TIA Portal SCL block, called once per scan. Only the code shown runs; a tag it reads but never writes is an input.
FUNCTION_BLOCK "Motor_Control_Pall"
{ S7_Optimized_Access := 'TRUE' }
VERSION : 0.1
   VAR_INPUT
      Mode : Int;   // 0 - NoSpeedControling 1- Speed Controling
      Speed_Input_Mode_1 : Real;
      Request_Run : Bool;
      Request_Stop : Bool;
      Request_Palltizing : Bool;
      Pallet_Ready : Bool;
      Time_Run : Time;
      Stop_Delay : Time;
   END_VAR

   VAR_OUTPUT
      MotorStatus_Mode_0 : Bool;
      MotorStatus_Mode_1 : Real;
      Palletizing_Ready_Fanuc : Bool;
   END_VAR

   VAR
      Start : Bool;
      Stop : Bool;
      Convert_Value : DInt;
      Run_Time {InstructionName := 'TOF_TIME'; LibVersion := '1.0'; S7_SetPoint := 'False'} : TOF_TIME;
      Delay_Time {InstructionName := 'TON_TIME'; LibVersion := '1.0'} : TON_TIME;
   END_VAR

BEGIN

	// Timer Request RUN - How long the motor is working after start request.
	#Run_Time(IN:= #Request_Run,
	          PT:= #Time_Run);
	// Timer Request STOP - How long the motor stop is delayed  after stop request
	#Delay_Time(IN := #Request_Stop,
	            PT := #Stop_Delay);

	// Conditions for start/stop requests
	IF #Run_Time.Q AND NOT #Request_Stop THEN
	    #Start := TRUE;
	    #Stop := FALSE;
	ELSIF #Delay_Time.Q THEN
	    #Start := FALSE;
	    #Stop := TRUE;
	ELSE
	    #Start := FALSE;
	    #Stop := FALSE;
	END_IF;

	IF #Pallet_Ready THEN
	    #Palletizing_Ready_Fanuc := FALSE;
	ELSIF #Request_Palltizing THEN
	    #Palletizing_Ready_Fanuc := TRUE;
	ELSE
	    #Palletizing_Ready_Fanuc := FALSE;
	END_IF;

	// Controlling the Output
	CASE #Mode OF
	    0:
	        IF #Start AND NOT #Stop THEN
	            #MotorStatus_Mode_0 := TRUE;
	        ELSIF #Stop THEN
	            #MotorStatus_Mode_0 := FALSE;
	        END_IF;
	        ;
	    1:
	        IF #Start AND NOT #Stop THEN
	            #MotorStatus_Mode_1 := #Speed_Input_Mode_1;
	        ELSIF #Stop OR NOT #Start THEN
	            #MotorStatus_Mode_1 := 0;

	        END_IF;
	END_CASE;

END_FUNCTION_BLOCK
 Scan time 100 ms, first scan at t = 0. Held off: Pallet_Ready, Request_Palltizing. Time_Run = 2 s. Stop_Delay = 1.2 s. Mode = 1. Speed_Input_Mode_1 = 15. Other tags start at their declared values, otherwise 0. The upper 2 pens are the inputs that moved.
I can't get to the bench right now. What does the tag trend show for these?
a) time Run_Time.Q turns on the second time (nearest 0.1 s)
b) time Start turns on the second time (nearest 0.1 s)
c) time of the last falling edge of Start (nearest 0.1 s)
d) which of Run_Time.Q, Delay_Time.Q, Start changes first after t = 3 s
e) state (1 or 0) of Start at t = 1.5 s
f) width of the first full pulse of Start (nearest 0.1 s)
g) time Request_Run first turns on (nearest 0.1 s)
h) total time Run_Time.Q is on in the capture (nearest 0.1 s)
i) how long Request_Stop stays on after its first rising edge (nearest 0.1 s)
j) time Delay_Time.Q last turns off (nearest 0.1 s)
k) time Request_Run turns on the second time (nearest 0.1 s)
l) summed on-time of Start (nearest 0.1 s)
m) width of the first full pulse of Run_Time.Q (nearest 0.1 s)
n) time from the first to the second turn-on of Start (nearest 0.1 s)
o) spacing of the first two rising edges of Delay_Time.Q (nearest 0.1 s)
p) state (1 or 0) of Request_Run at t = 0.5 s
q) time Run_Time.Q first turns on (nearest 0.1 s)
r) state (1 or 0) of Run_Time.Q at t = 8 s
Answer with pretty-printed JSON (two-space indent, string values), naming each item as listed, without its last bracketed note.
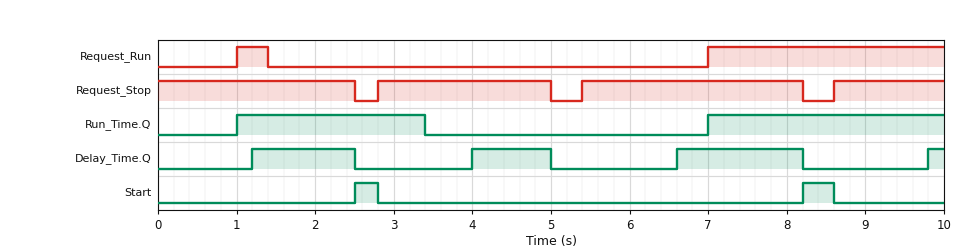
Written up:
{
  "time Run_Time.Q turns on the second time": "7.0 s",
  "time Start turns on the second time": "8.2 s",
  "time of the last falling edge of Start": "8.6 s",
  "which of Run_Time.Q, Delay_Time.Q, Start changes first after t = 3 s": "Run_Time.Q",
  "state (1 or 0) of Start at t = 1.5 s": "0",
  "width of the first full pulse of Start": "0.3 s",
  "time Request_Run first turns on": "1.0 s",
  "total time Run_Time.Q is on in the capture": "5.4 s",
  "how long Request_Stop stays on after its first rising edge": "2.2 s",
  "time Delay_Time.Q last turns off": "8.2 s",
  "time Request_Run turns on the second time": "7.0 s",
  "summed on-time of Start": "0.7 s",
  "width of the first full pulse of Run_Time.Q": "2.4 s",
  "time from the first to the second turn-on of Start": "5.7 s",
  "spacing of the first two rising edges of Delay_Time.Q": "2.8 s",
  "state (1 or 0) of Request_Run at t = 0.5 s": "0",
  "time Run_Time.Q first turns on": "1.0 s",
  "state (1 or 0) of Run_Time.Q at t = 8 s": "1"
}
